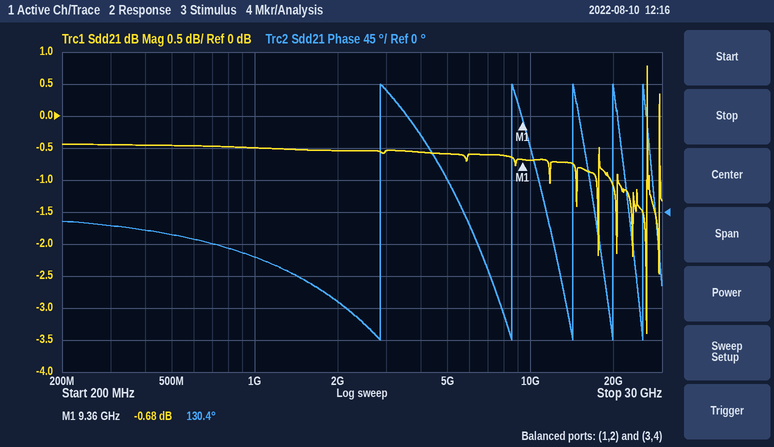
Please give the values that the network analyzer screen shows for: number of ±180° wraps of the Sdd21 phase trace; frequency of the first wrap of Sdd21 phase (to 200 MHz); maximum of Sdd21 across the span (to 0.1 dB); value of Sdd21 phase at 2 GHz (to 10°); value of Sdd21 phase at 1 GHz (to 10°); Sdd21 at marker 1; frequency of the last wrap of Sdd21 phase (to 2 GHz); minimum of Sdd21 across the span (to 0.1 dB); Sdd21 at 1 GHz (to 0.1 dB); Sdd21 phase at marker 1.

5
2.8 GHz
0.8 dB
-130°
-60°
-0.68 dB
26 GHz
-3.4 dB
-0.5 dB
130.4°
